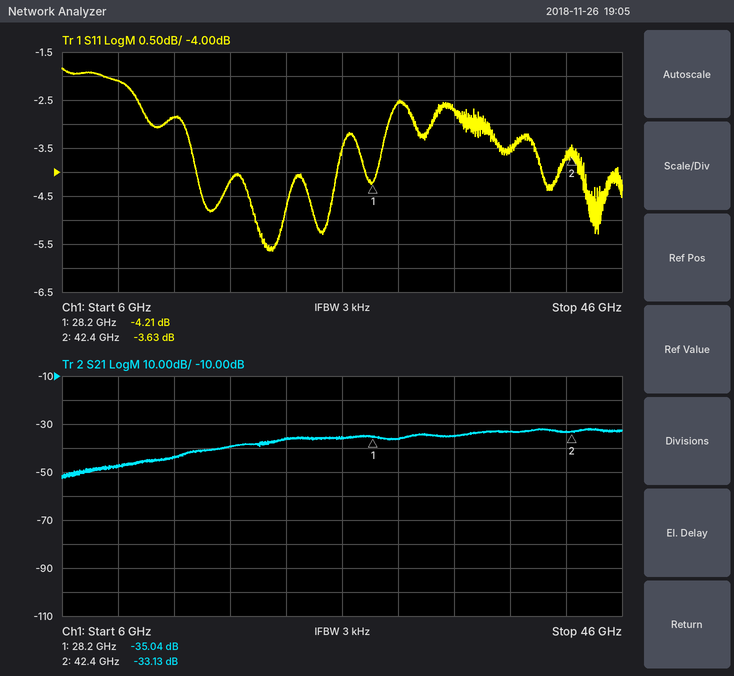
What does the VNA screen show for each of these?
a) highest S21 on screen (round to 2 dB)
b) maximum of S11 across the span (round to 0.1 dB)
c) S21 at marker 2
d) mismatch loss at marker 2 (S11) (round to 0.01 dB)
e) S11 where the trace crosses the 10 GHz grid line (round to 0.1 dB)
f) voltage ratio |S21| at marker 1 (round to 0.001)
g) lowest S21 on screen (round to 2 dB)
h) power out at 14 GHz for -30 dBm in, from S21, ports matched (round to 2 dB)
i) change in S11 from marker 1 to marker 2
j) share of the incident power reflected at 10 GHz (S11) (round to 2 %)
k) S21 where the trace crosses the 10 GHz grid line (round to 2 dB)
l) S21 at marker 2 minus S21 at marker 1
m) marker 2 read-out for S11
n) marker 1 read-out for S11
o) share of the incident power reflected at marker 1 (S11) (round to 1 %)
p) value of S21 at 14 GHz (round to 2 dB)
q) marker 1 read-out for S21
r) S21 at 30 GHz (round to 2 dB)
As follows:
-32 dB
-1.8 dB
-33.13 dB
2.47 dB
-2.1 dB
0.018
-52 dB
-74 dBm
0.58 dB
62 %
-48 dB
1.91 dB
-3.63 dB
-4.21 dB
38 %
-44 dB
-35.04 dB
-36 dB
